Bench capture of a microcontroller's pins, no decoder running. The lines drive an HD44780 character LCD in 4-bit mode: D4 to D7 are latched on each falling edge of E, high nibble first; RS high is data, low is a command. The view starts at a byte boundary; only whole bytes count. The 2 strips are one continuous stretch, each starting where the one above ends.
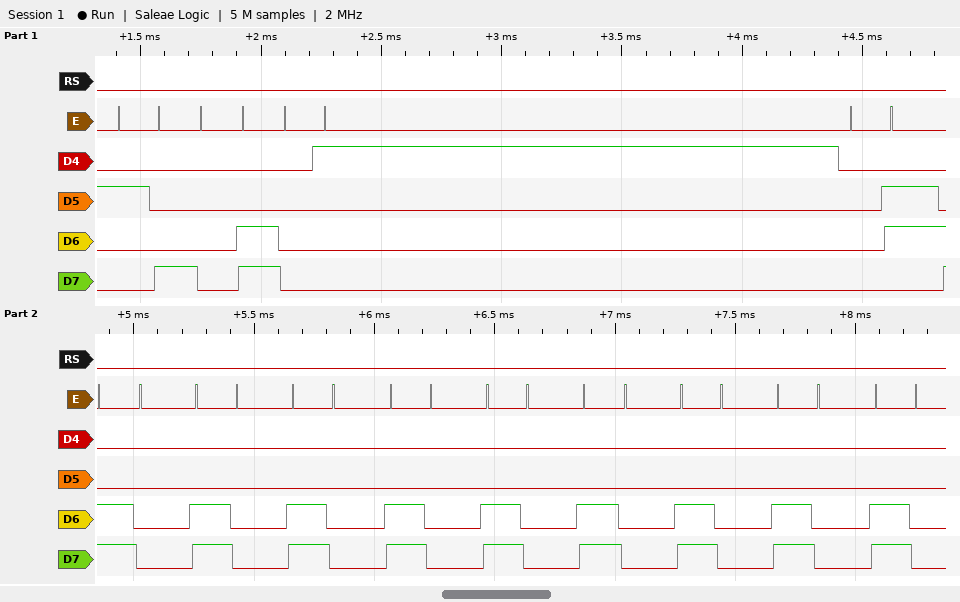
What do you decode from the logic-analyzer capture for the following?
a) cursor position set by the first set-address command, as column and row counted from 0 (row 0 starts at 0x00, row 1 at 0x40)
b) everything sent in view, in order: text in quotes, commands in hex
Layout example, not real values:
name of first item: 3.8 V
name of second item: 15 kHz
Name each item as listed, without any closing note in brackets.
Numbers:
cursor position set by the first set-address command, as column and row counted from 0: column 0, row 1
everything sent in view, in order: text in quotes, commands in hex: 0x28 0x0C 0x01 0x06 0xC0 0xC0 0xC0 0xC0 0xC0 0xC0 0xC0 0xC0 0xC0
